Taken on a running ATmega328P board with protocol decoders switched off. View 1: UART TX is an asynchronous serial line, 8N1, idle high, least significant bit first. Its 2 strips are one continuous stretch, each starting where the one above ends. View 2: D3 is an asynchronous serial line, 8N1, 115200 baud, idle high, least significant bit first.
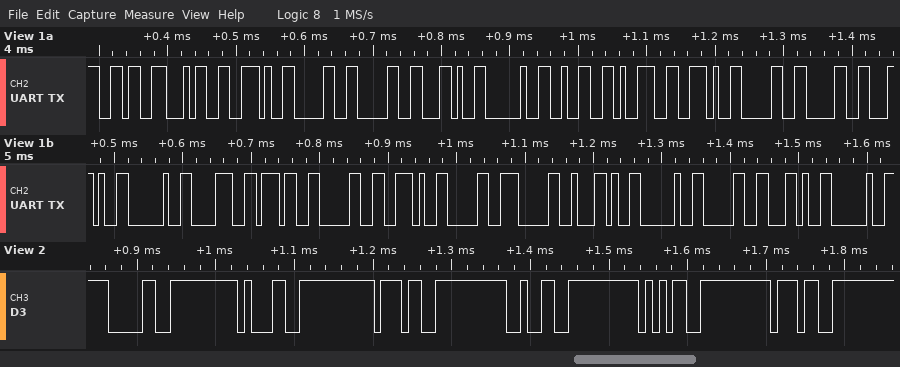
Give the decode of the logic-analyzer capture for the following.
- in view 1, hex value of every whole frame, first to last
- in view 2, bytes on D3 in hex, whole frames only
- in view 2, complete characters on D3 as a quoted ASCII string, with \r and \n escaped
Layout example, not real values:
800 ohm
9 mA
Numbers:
36 34 2E 30 30 2C 20 32 39 2E 30 30 2C 20 38 37 30 2E 30 30 2C 20 30 2C 20
30 31 37 32 35 37
"017257"
